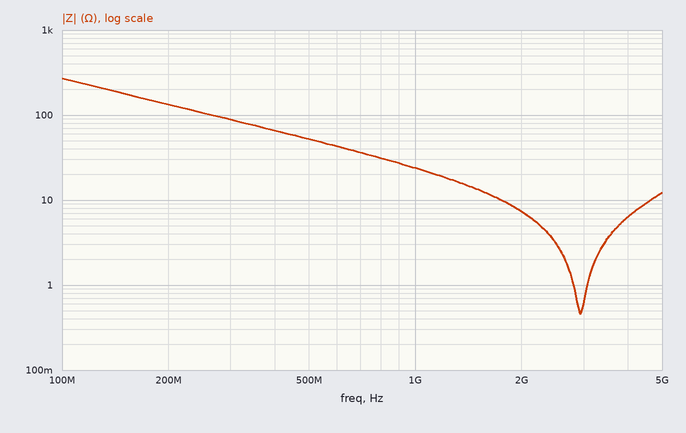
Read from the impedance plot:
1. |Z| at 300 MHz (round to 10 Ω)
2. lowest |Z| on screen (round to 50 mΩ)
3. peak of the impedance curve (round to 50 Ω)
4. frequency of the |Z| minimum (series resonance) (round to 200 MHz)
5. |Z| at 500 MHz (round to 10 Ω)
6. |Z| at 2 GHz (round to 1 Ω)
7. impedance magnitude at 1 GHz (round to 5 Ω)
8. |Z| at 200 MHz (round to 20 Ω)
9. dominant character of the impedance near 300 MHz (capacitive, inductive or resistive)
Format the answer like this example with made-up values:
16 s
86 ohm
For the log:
90 Ω
450 mΩ
250 Ω
3.0 GHz
50 Ω
7 Ω
25 Ω
140 Ω
capacitive
